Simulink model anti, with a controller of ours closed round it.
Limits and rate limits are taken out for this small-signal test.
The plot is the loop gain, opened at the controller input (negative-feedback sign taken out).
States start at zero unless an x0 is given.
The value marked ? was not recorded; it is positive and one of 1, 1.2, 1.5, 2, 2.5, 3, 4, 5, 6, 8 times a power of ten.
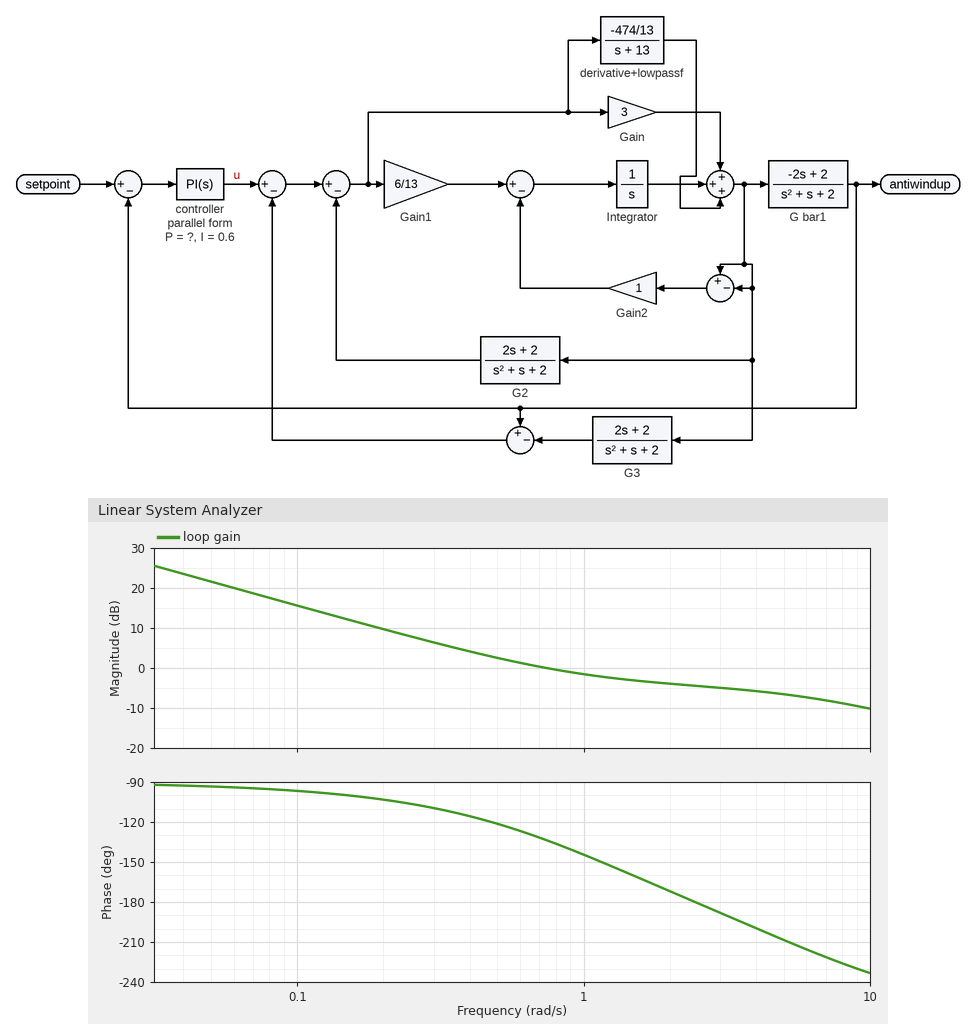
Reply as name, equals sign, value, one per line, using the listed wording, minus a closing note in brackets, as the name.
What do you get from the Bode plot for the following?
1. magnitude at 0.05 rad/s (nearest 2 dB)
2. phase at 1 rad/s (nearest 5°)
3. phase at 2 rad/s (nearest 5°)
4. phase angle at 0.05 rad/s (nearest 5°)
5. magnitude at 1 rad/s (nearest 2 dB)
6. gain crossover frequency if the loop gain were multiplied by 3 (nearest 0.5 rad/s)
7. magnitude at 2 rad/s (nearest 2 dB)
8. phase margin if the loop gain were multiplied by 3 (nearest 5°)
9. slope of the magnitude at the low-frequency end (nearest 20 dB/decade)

magnitude at 0.05 rad/s = 22 dB
phase at 1 rad/s = -145°
phase at 2 rad/s = -170°
phase angle at 0.05 rad/s = -95°
magnitude at 1 rad/s = -2 dB
gain crossover frequency if the loop gain were multiplied by 3 = 9.0 rad/s
magnitude at 2 rad/s = -4 dB
phase margin if the loop gain were multiplied by 3 = -50°
slope of the magnitude at the low-frequency end = -20 dB/decade
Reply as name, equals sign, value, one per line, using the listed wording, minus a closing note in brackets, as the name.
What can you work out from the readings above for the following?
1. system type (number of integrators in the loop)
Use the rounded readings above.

system type = 1
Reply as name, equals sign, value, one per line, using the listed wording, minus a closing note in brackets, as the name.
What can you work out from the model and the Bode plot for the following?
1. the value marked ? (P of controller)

the value marked ? = 0.6
